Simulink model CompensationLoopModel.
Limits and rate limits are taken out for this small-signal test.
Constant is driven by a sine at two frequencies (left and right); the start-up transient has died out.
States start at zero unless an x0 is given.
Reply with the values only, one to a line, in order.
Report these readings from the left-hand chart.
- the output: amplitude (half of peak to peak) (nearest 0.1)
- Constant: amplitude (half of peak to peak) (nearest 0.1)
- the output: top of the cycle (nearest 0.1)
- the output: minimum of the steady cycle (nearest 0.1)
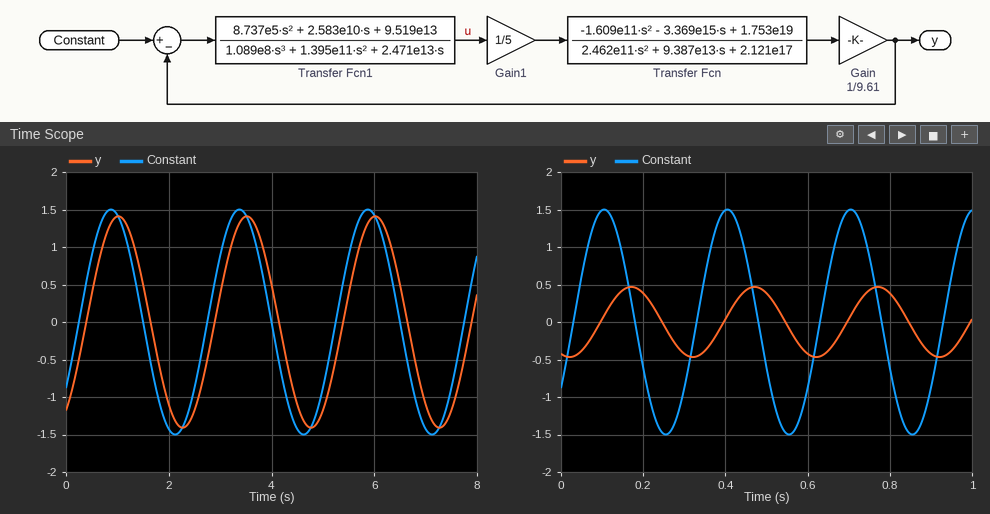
1.4
1.5
1.4
-1.4
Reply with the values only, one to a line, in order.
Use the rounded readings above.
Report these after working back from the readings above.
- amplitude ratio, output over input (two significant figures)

0.93
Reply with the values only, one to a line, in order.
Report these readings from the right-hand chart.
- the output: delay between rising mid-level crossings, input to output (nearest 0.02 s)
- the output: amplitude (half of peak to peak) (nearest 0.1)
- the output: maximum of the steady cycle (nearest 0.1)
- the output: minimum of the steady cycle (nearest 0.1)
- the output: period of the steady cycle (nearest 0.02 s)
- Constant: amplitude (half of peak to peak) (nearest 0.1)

0.06 s
0.5
0.5
-0.5
0.30 s
1.5
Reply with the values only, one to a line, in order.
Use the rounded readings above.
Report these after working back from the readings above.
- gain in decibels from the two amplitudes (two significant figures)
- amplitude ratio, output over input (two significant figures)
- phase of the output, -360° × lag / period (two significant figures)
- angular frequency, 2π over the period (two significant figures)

-9.5 dB
0.33
-72°
21 rad/s
